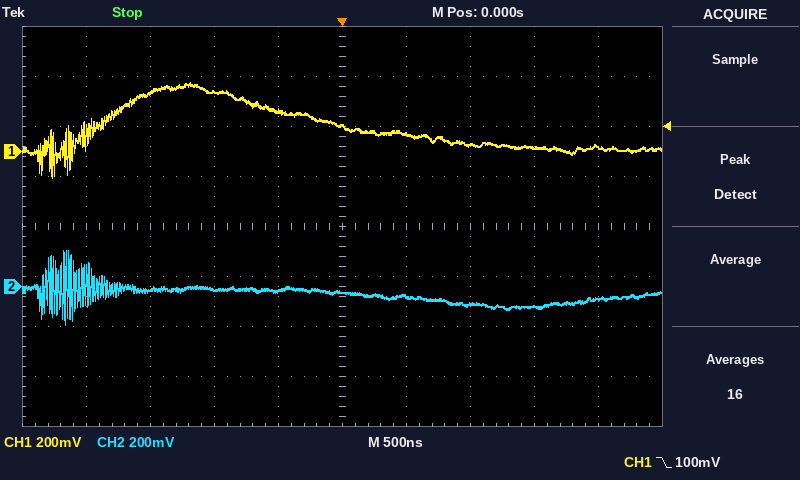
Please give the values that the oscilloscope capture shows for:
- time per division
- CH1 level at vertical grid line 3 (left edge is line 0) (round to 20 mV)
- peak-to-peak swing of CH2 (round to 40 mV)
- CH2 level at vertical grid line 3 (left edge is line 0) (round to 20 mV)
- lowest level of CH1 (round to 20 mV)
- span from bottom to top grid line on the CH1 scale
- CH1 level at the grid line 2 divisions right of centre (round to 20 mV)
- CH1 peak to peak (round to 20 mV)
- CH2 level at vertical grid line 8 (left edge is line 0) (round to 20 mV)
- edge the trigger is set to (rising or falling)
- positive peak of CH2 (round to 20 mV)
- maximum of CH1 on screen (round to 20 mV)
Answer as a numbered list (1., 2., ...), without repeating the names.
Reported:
1. 500 ns
2. 240 mV
3. 280 mV
4. -20 mV
5. -100 mV
6. 1.6 V
7. 20 mV
8. 380 mV
9. -80 mV
10. falling
11. 140 mV
12. 280 mV
